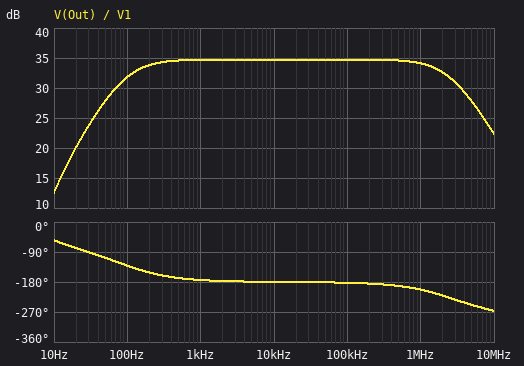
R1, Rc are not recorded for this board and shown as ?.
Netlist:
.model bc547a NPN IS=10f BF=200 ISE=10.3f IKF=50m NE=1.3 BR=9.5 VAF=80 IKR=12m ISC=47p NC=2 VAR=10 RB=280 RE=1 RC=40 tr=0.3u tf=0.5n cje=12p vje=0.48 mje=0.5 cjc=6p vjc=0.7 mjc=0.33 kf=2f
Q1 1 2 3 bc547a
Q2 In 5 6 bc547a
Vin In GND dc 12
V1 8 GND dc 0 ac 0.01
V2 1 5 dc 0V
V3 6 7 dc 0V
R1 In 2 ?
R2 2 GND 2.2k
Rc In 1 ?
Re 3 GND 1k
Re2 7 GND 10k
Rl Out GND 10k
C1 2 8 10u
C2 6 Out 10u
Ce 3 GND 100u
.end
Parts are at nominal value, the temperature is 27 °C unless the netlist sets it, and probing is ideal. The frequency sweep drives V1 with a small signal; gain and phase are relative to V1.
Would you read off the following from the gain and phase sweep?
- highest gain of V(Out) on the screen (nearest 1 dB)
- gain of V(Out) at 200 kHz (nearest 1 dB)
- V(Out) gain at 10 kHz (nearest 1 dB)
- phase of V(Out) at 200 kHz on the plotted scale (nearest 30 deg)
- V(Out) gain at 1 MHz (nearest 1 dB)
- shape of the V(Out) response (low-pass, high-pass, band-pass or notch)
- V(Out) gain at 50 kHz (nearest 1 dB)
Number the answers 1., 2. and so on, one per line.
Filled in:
1. 35 dB
2. 35 dB
3. 35 dB
4. -180 deg
5. 34 dB
6. band-pass
7. 35 dB
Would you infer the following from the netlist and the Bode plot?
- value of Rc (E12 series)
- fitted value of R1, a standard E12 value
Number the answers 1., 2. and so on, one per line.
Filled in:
1. 1 kΩ
2. 8.2 kΩ
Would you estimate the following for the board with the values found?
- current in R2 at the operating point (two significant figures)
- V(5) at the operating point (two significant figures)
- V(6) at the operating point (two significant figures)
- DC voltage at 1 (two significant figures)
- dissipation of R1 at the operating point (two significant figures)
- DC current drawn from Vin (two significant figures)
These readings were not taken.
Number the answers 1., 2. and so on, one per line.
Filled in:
1. 1.1 mA
2. 10 V
3. 9.5 V
4. 10 V
5. 11 mW
6. 3.9 mA
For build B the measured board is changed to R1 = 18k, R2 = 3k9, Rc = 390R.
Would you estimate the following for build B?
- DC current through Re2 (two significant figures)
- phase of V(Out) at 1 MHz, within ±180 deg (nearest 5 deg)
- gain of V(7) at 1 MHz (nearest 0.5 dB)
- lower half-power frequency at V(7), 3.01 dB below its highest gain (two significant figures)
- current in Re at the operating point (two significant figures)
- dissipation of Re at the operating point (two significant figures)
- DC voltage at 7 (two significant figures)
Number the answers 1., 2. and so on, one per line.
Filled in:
1. 1.1 mA
2. 170 deg
3. 25.0 dB
4. 81 Hz
5. 1.4 mA
6. 2.1 mW
7. 11 V
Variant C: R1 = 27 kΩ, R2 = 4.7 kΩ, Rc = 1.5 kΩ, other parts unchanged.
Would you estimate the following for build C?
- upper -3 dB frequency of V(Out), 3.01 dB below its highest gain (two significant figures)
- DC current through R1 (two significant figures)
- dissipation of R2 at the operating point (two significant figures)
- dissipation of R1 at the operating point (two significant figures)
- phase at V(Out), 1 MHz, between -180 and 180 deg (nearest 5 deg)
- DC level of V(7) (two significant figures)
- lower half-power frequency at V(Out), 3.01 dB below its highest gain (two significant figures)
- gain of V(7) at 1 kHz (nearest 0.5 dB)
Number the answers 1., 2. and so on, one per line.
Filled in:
1. 2.6 MHz
2. 380 µA
3. 650 µW
4. 3.9 mW
5. 160 deg
6. 9.7 V
7. 63 Hz
8. 34.5 dB
